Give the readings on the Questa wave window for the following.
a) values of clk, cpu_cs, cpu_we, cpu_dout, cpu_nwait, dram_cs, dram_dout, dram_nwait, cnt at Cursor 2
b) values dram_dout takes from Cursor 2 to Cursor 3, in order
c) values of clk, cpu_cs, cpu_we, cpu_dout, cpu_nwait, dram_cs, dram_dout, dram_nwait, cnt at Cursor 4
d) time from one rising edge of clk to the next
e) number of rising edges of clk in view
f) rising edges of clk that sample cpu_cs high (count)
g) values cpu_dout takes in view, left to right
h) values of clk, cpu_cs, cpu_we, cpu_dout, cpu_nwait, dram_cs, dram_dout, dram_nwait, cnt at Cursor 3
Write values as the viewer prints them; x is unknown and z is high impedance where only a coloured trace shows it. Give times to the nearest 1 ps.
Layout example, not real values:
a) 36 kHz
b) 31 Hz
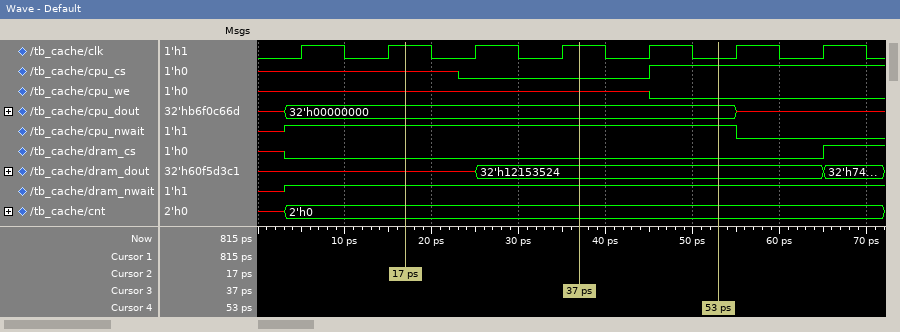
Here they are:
a) clk=1, cpu_cs=x, cpu_we=x, cpu_dout=32'h00000000, cpu_nwait=1, dram_cs=0, dram_dout=x, dram_nwait=1, cnt=2'h0
b) x, 32'h12153524
c) clk=0, cpu_cs=1, cpu_we=0, cpu_dout=32'h00000000, cpu_nwait=1, dram_cs=0, dram_dout=32'h12153524, dram_nwait=1, cnt=2'h0
d) 10 ps
e) 7
f) 2
g) x, 32'h00000000, x
h) clk=1, cpu_cs=0, cpu_we=x, cpu_dout=32'h00000000, cpu_nwait=1, dram_cs=0, dram_dout=32'h12153524, dram_nwait=1, cnt=2'h0
